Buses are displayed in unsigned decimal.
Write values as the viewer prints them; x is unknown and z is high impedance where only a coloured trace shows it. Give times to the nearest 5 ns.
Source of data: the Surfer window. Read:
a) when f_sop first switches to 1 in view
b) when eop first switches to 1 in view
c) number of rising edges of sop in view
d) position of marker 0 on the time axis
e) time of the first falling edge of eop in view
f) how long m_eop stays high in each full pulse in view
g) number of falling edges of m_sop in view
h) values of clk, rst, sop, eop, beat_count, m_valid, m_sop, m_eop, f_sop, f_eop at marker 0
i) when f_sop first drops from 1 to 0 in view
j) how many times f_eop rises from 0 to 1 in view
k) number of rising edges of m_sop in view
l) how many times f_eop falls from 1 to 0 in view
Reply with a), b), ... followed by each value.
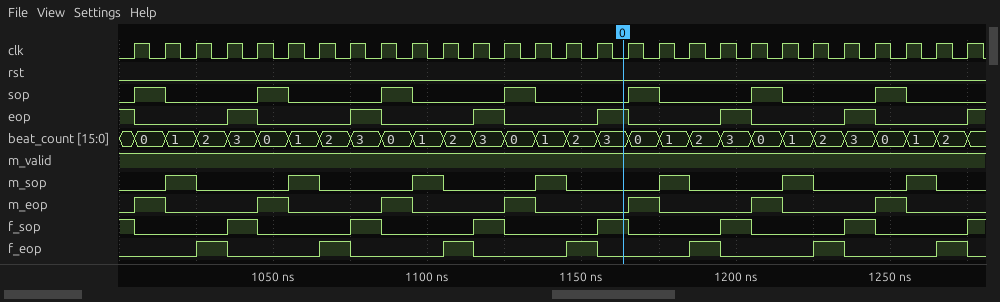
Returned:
a) 1035 ns
b) 1035 ns
c) 7
d) 1165 ns
e) 1005 ns
f) 10 ns, 10 ns, 10 ns, 10 ns, 10 ns, 10 ns, 10 ns
g) 7
h) clk=0, rst=0, sop=0, eop=1, beat_count=3, m_valid=1, m_sop=0, m_eop=0, f_sop=1, f_eop=0
i) 1005 ns
j) 7
k) 7
l) 7
